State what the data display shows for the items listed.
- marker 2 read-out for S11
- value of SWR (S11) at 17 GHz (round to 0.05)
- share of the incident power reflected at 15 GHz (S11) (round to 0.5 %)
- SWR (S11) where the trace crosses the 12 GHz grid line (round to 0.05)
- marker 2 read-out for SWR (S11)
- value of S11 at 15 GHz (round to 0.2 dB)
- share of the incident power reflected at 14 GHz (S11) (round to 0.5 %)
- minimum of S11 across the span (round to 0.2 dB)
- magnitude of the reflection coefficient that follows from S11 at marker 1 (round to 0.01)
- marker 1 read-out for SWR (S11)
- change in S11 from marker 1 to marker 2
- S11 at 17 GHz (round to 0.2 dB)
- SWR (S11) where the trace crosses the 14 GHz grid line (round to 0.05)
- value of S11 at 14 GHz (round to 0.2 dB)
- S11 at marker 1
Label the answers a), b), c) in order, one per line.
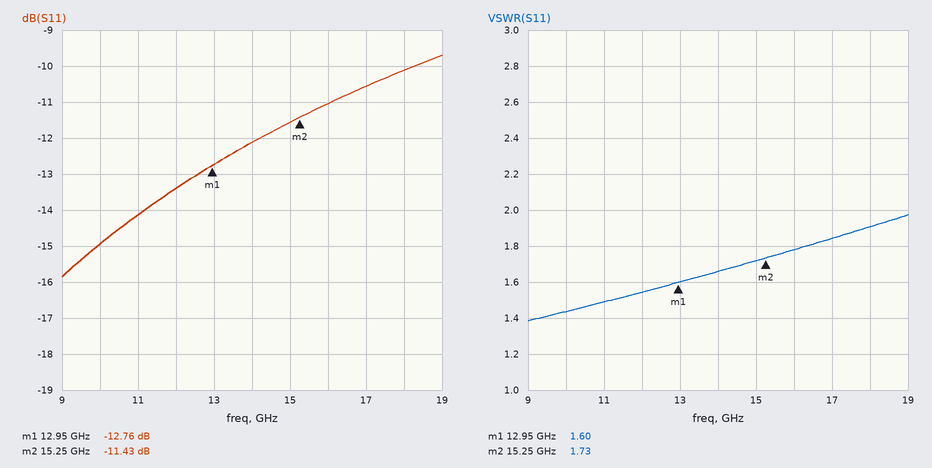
a) -11.43 dB
b) 1.85
c) 7.0 %
d) 1.55
e) 1.73
f) -11.6 dB
g) 6.0 %
h) -15.8 dB
i) 0.23
j) 1.60
k) 1.33 dB
l) -10.6 dB
m) 1.65
n) -12.2 dB
o) -12.76 dB
